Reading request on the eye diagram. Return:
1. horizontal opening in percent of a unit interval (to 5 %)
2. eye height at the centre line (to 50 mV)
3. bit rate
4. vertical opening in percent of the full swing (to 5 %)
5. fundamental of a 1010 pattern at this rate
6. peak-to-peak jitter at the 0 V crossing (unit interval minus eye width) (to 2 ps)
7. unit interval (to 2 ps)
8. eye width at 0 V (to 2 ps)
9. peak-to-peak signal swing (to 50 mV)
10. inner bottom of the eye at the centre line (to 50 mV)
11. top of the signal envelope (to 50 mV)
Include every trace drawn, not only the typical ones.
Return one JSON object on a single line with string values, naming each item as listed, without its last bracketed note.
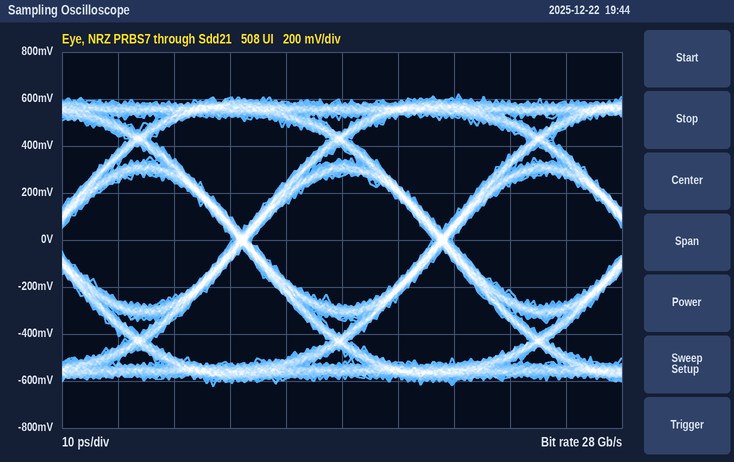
{"horizontal opening in percent of a unit interval": "90 %", "eye height at the centre line": "550 mV", "bit rate": "28 Gb/s", "vertical opening in percent of the full swing": "45 %", "fundamental of a 1010 pattern at this rate": "14 GHz", "peak-to-peak jitter at the 0 V crossing (unit interval minus eye width)": "4 ps", "unit interval": "36 ps", "eye width at 0 V": "32 ps", "peak-to-peak signal swing": "1.25 V", "inner bottom of the eye at the centre line": "-300 mV", "top of the signal envelope": "600 mV"}
